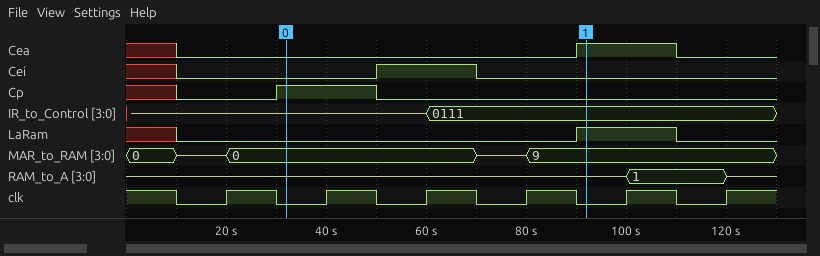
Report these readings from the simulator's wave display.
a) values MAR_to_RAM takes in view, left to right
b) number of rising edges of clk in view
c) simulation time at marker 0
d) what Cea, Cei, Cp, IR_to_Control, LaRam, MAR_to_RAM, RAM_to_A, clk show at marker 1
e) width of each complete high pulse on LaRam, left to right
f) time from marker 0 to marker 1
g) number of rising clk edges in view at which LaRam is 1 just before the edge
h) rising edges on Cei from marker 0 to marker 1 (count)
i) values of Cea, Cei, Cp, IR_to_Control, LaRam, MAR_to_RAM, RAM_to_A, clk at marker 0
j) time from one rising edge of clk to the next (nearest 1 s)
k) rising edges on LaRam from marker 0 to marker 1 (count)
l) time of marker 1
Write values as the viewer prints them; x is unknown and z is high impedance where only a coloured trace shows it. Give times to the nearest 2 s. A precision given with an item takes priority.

0, z, 0, z, 9
6
32 s
Cea=1, Cei=0, Cp=0, IR_to_Control=0111, LaRam=1, MAR_to_RAM=9, RAM_to_A=z, clk=0
20 s
60 s
1
1
Cea=0, Cei=0, Cp=1, IR_to_Control=z, LaRam=0, MAR_to_RAM=0, RAM_to_A=z, clk=0
20 s
1
92 s
